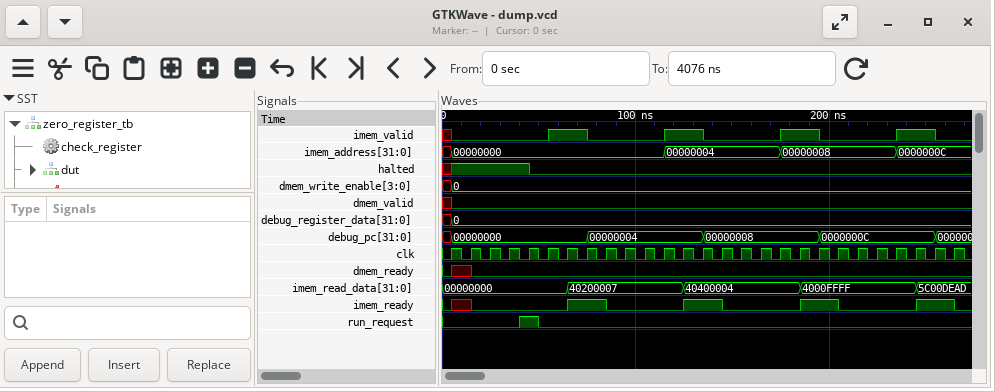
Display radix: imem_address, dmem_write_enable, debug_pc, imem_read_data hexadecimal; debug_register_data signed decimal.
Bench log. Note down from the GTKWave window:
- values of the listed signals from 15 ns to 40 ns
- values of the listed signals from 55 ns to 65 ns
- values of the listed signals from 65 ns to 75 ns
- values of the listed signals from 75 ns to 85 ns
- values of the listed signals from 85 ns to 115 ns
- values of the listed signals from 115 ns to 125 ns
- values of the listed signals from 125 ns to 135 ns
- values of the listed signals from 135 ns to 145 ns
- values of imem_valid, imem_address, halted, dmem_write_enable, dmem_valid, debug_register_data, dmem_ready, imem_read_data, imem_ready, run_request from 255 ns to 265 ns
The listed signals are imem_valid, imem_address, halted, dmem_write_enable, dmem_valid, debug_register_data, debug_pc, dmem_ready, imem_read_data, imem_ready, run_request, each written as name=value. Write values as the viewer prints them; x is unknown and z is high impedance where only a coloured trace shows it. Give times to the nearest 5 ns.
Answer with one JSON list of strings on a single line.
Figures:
["imem_valid=0, imem_address=00000000, halted=1, dmem_write_enable=0, dmem_valid=0, debug_register_data=0, debug_pc=00000000, dmem_ready=0, imem_read_data=00000000, imem_ready=0, run_request=0", "imem_valid=1, imem_address=00000000, halted=0, dmem_write_enable=0, dmem_valid=0, debug_register_data=0, debug_pc=00000000, dmem_ready=0, imem_read_data=00000000, imem_ready=0, run_request=0", "imem_valid=1, imem_address=00000000, halted=0, dmem_write_enable=0, dmem_valid=0, debug_register_data=0, debug_pc=00000000, dmem_ready=0, imem_read_data=40200007, imem_ready=1, run_request=0", "imem_valid=0, imem_address=00000000, halted=0, dmem_write_enable=0, dmem_valid=0, debug_register_data=0, debug_pc=00000004, dmem_ready=0, imem_read_data=40200007, imem_ready=1, run_request=0", "imem_valid=0, imem_address=00000000, halted=0, dmem_write_enable=0, dmem_valid=0, debug_register_data=0, debug_pc=00000004, dmem_ready=0, imem_read_data=40200007, imem_ready=0, run_request=0", "imem_valid=1, imem_address=00000004, halted=0, dmem_write_enable=0, dmem_valid=0, debug_register_data=0, debug_pc=00000004, dmem_ready=0, imem_read_data=40200007, imem_ready=0, run_request=0", "imem_valid=1, imem_address=00000004, halted=0, dmem_write_enable=0, dmem_valid=0, debug_register_data=0, debug_pc=00000004, dmem_ready=0, imem_read_data=40400004, imem_ready=1, run_request=0", "imem_valid=0, imem_address=00000004, halted=0, dmem_write_enable=0, dmem_valid=0, debug_register_data=0, debug_pc=00000008, dmem_ready=0, imem_read_data=40400004, imem_ready=1, run_request=0", "imem_valid=0, imem_address=0000000C, halted=0, dmem_write_enable=0, dmem_valid=0, debug_register_data=0, dmem_ready=0, imem_read_data=5C00DEAD, imem_ready=1, run_request=0"]
